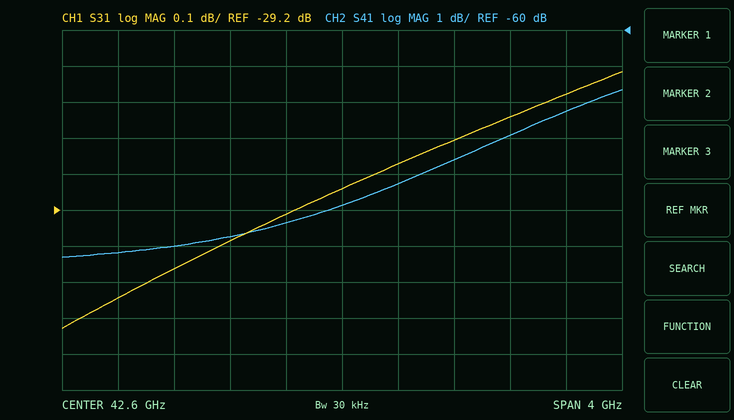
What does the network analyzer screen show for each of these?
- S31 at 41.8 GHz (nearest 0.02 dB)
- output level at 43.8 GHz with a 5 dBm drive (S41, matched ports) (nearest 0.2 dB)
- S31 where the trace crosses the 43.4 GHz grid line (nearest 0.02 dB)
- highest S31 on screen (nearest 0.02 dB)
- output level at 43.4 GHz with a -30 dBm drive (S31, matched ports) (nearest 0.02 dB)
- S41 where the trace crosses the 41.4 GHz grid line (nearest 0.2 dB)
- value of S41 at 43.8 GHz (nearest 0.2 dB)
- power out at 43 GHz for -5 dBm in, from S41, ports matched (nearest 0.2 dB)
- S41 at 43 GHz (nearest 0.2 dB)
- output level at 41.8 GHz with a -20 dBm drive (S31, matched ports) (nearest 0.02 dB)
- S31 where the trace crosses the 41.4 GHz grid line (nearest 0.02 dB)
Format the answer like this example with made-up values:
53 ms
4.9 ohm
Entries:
-29.28 dB
-58.0 dBm
-29.00 dB
-28.82 dB
-59.00 dBm
-66.0 dB
-63.0 dB
-69.2 dBm
-64.2 dB
-49.28 dBm
-29.36 dB
